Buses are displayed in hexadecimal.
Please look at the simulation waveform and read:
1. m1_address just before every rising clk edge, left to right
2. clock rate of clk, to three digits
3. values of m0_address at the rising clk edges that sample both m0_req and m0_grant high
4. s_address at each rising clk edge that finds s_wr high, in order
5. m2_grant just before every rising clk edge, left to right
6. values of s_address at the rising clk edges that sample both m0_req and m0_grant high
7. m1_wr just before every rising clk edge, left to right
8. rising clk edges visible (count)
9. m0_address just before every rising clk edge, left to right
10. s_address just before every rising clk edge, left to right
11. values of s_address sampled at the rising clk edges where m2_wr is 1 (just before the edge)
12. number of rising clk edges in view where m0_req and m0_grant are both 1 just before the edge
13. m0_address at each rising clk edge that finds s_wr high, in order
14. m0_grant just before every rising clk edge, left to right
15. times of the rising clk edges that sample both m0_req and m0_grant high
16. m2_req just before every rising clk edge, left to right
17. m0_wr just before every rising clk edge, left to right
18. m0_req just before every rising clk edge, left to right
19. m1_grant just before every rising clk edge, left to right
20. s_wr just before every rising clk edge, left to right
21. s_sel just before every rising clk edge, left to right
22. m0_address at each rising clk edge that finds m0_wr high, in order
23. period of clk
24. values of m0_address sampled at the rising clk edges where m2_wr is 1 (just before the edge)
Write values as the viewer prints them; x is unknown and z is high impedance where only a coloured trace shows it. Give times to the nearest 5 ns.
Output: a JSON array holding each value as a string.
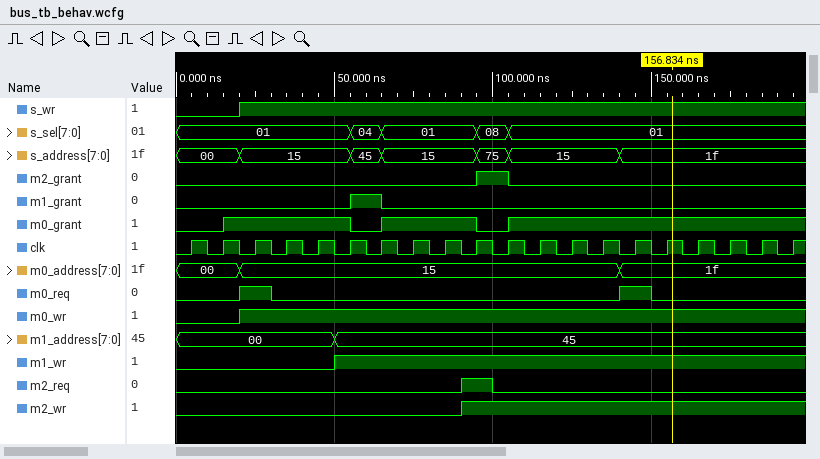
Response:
["00, 00, 00, 00, 00, 45, 45, 45, 45, 45, 45, 45, 45, 45, 45, 45, 45, 45, 45, 45", "100 MHz", "15, 1f", "15, 15, 15, 15, 45, 15, 15, 15, 75, 15, 15, 15, 1f, 1f, 1f, 1f, 1f, 1f", "0 0 0 0 0 0 0 0 0 0 1 0 0 0 0 0 0 0 0 0", "15, 1f", "0 0 0 0 0 1 1 1 1 1 1 1 1 1 1 1 1 1 1 1", "20", "00, 00, 15, 15, 15, 15, 15, 15, 15, 15, 15, 15, 15, 15, 1f, 1f, 1f, 1f, 1f, 1f", "00, 00, 15, 15, 15, 15, 45, 15, 15, 15, 75, 15, 15, 15, 1f, 1f, 1f, 1f, 1f, 1f", "15, 75, 15, 15, 15, 1f, 1f, 1f, 1f, 1f, 1f", "2", "15, 15, 15, 15, 15, 15, 15, 15, 15, 15, 15, 15, 1f, 1f, 1f, 1f, 1f, 1f", "0 0 1 1 1 1 0 1 1 1 0 1 1 1 1 1 1 1 1 1", "25 ns, 145 ns", "0 0 0 0 0 0 0 0 0 1 0 0 0 0 0 0 0 0 0 0", "0 0 1 1 1 1 1 1 1 1 1 1 1 1 1 1 1 1 1 1", "0 0 1 0 0 0 0 0 0 0 0 0 0 0 1 0 0 0 0 0", "0 0 0 0 0 0 1 0 0 0 0 0 0 0 0 0 0 0 0 0", "0 0 1 1 1 1 1 1 1 1 1 1 1 1 1 1 1 1 1 1", "01, 01, 01, 01, 01, 01, 04, 01, 01, 01, 08, 01, 01, 01, 01, 01, 01, 01, 01, 01", "15, 15, 15, 15, 15, 15, 15, 15, 15, 15, 15, 15, 1f, 1f, 1f, 1f, 1f, 1f", "10 ns", "15, 15, 15, 15, 15, 1f, 1f, 1f, 1f, 1f, 1f"]
